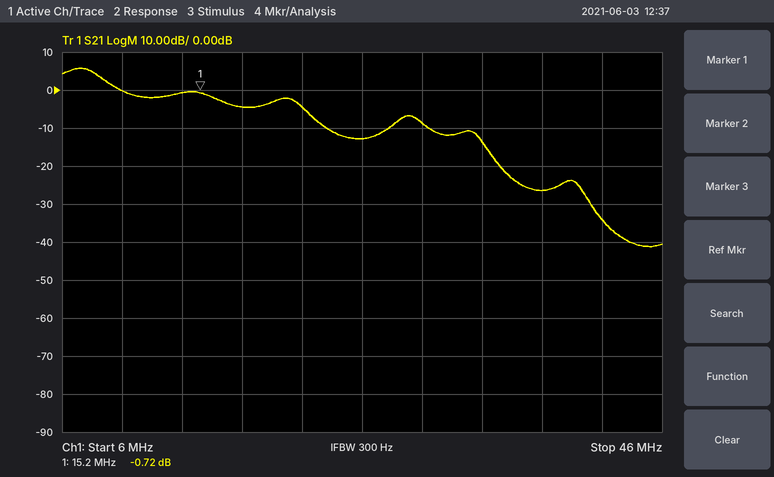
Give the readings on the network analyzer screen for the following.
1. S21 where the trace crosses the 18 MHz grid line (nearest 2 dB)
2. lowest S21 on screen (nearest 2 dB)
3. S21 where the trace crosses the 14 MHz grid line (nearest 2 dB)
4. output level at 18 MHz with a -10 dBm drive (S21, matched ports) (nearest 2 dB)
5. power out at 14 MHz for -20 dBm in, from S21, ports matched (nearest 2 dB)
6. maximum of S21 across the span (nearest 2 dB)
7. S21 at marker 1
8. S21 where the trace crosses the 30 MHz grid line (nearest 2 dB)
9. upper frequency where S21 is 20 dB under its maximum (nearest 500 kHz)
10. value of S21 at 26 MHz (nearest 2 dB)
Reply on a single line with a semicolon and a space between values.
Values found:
-4 dB; -42 dB; 0 dB; -14 dBm; -20 dBm; 6 dB; -0.72 dB; -8 dB; 34.0 MHz; -12 dB
